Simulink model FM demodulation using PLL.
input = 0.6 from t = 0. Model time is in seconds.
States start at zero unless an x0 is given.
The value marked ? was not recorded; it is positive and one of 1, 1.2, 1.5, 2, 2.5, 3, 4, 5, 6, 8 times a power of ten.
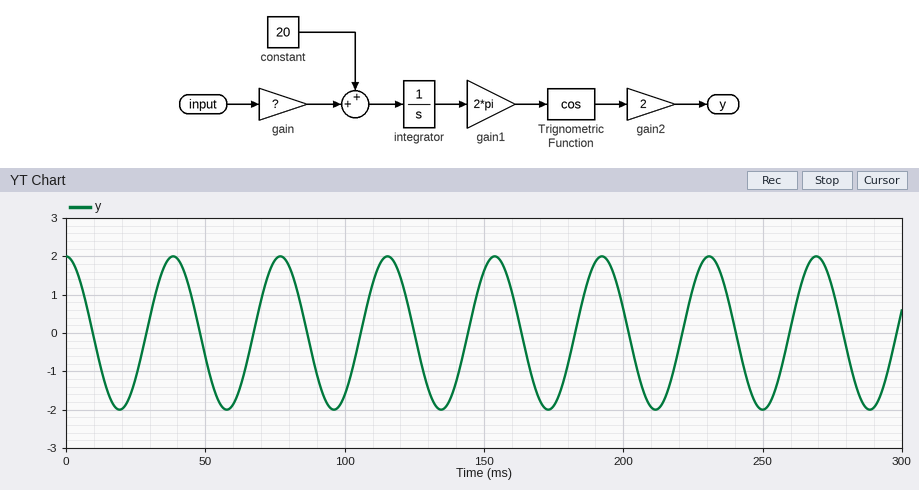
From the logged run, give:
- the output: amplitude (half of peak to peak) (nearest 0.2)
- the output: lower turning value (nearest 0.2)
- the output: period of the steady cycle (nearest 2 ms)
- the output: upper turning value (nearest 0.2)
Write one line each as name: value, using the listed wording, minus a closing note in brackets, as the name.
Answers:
the output: amplitude (half of peak to peak): 2.0
the output: lower turning value: -2.0
the output: period of the steady cycle: 38 ms
the output: upper turning value: 2.0
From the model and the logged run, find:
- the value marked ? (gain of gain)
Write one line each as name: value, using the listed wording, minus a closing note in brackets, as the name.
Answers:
the value marked ?: 10
